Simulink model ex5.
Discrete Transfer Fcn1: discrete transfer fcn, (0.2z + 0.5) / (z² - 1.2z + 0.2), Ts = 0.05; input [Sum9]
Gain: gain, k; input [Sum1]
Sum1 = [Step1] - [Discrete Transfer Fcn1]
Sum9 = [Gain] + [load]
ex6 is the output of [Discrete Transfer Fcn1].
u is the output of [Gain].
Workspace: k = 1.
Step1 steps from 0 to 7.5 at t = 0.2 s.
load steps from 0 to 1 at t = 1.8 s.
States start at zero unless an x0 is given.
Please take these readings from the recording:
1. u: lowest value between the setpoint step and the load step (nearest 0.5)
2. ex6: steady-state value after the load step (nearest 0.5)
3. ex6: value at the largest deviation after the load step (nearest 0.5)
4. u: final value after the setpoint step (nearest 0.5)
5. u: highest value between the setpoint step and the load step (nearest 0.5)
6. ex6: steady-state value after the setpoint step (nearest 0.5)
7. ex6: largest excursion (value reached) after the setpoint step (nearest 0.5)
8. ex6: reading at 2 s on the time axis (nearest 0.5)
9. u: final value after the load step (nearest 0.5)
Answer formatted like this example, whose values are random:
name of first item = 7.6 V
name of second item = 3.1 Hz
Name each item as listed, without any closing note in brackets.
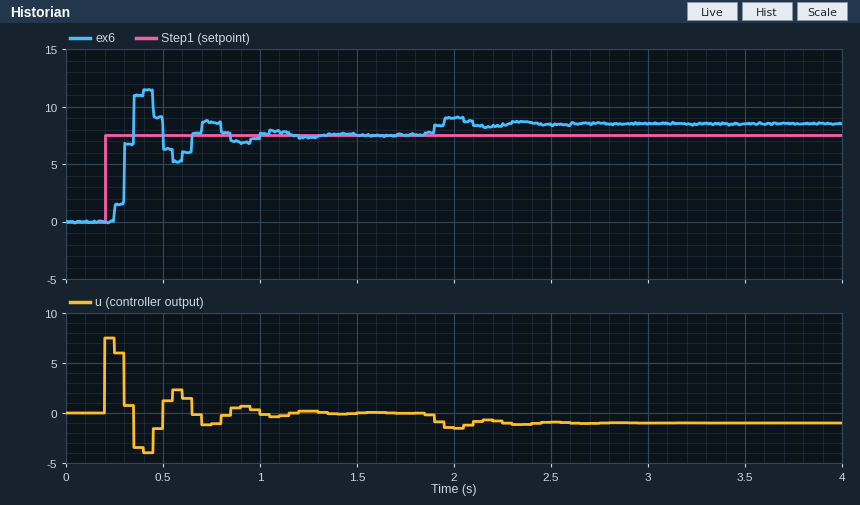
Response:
u: lowest value between the setpoint step and the load step = -4.0
ex6: steady-state value after the load step = 8.5
ex6: value at the largest deviation after the load step = 9.0
u: final value after the setpoint step = 0.0
u: highest value between the setpoint step and the load step = 7.5
ex6: steady-state value after the setpoint step = 7.5
ex6: largest excursion (value reached) after the setpoint step = 11.5
ex6: reading at 2 s on the time axis = 9.0
u: final value after the load step = -1.0
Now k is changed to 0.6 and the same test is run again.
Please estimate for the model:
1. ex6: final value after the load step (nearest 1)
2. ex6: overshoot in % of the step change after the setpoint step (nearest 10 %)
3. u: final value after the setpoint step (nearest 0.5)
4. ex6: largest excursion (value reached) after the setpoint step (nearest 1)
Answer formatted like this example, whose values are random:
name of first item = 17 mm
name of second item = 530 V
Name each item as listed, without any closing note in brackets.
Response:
ex6: final value after the load step = 9
ex6: overshoot in % of the step change after the setpoint step = 20 %
u: final value after the setpoint step = 0.0
ex6: largest excursion (value reached) after the setpoint step = 9
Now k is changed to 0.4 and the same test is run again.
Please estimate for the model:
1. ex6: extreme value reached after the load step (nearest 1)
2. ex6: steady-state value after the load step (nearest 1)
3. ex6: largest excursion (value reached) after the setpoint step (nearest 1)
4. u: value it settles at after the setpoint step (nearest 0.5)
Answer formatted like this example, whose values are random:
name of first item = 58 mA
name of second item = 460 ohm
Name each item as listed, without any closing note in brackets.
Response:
ex6: extreme value reached after the load step = 10
ex6: steady-state value after the load step = 10
ex6: largest excursion (value reached) after the setpoint step = 8
u: value it settles at after the setpoint step = 0.0
